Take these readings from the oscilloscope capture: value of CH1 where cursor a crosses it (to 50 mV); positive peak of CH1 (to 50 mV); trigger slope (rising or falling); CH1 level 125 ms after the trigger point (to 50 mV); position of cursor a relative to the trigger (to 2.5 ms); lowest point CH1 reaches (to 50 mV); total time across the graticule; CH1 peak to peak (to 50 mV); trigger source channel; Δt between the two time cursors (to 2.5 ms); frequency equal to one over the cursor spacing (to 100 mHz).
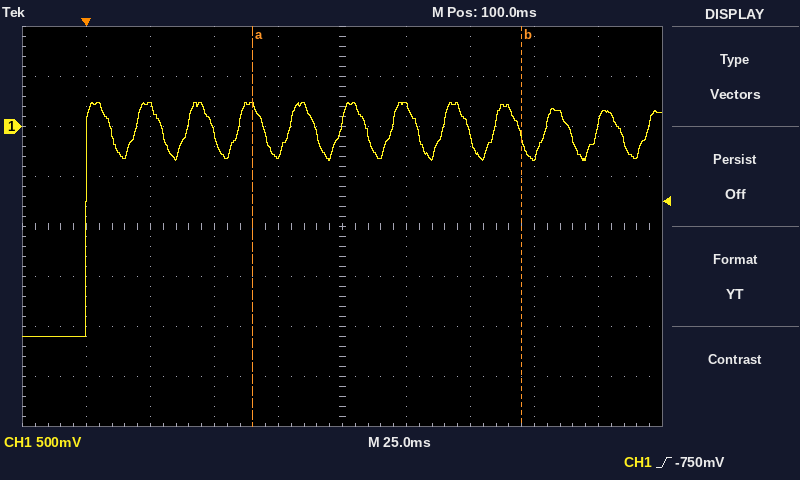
200 mV
250 mV
rising
200 mV
+65.0 ms
-2.10 V
250 ms
2.35 V
CH1
105.0 ms
9.5 Hz
